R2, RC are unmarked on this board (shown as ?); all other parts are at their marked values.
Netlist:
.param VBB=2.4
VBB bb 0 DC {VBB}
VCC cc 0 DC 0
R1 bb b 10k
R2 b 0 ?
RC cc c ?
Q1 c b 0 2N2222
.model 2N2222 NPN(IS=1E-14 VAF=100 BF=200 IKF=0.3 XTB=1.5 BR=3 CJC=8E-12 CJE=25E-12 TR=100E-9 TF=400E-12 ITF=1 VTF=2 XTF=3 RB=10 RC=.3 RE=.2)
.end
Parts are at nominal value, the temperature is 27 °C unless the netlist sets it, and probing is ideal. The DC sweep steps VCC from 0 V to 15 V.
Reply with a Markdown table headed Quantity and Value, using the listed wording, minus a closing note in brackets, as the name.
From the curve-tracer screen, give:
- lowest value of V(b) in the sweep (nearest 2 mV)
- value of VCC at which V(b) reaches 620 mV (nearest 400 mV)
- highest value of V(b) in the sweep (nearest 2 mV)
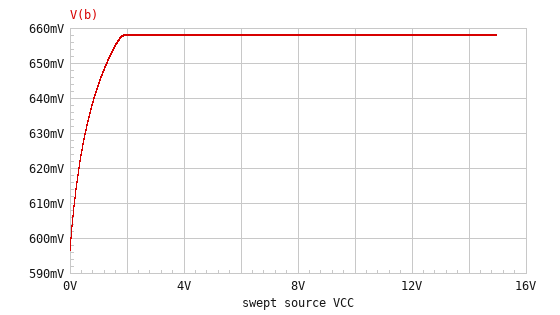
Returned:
| Quantity | Value |
|---|---|
| lowest value of V(b) in the sweep | 596 mV |
| value of VCC at which V(b) reaches 620 mV | 400 mV |
| highest value of V(b) in the sweep | 658 mV |
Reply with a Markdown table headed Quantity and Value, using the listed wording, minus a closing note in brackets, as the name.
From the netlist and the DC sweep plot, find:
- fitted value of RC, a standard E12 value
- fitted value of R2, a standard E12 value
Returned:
| Quantity | Value |
|---|---|
| fitted value of RC, a standard E12 value | 1.5 kΩ |
| fitted value of R2, a standard E12 value | 3.9 kΩ |
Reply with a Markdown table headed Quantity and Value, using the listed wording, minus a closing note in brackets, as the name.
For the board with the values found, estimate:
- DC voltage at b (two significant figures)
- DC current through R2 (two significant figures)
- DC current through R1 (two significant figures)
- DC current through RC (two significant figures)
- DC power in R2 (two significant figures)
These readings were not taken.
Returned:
| Quantity | Value |
|---|---|
| DC voltage at b | 600 mV |
| DC current through R2 | 150 µA |
| DC current through R1 | 180 µA |
| DC current through RC | 4.3 µA |
| DC power in R2 | 91 µW |
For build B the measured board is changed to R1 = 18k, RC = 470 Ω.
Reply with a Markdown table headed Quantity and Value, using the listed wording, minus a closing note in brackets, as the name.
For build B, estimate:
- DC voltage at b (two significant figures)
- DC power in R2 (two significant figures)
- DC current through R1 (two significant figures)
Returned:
| Quantity | Value |
|---|---|
| DC voltage at b | 430 mV |
| DC power in R2 | 47 µW |
| DC current through R1 | 110 µA |
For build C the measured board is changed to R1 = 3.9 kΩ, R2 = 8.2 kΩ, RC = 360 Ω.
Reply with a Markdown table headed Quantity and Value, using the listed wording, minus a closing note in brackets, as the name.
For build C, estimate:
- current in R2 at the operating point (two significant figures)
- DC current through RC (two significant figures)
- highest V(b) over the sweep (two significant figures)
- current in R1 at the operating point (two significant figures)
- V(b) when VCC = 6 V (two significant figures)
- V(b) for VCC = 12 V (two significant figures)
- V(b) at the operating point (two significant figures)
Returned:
| Quantity | Value |
|---|---|
| current in R2 at the operating point | 81 µA |
| DC current through RC | 20 µA |
| highest V(b) over the sweep | 770 mV |
| current in R1 at the operating point | 440 µA |
| V(b) when VCC = 6 V | 740 mV |
| V(b) for VCC = 12 V | 760 mV |
| V(b) at the operating point | 670 mV |
